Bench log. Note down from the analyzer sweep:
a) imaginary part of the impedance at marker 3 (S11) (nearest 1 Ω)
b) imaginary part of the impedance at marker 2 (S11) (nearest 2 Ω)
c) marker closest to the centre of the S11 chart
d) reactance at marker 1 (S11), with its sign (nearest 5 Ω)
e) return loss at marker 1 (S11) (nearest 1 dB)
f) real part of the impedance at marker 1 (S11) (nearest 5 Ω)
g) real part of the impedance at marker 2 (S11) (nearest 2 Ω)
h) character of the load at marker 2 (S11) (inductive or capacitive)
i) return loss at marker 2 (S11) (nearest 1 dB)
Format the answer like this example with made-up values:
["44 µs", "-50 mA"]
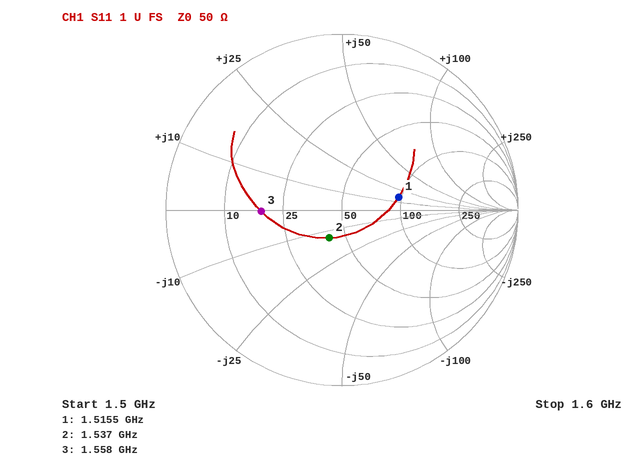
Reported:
["0 Ω", "-14 Ω", "marker 2", "+15 Ω", "10 dB", "95 Ω", "42 Ω", "capacitive", "15 dB"]
